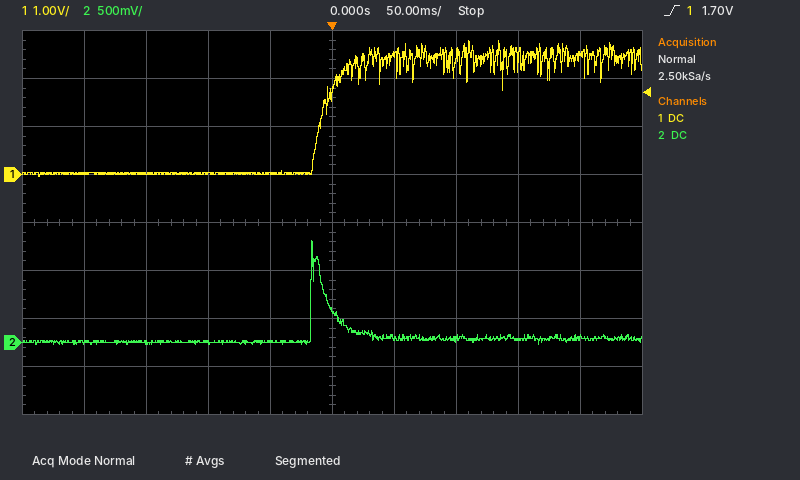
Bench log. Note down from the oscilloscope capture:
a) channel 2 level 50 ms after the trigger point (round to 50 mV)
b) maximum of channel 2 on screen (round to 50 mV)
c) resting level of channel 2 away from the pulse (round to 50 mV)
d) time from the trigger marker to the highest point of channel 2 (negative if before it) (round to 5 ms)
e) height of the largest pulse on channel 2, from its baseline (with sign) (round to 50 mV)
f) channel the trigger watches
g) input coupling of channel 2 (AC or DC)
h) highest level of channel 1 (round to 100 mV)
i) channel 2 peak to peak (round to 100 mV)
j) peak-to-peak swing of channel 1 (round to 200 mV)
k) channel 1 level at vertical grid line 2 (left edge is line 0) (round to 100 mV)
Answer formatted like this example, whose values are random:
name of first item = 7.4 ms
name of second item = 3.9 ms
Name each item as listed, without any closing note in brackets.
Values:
channel 2 level 50 ms after the trigger point = 50 mV
maximum of channel 2 on screen = 1.05 V
resting level of channel 2 away from the pulse = 0 mV
time from the trigger marker to the highest point of channel 2 (negative if before it) = -15 ms
height of the largest pulse on channel 2, from its baseline (with sign) = +1.05 V
channel the trigger watches = channel 1
input coupling of channel 2 = DC
highest level of channel 1 = 2.8 V
channel 2 peak to peak = 1.10 V
peak-to-peak swing of channel 1 = 2.8 V
channel 1 level at vertical grid line 2 (left edge is line 0) = 0.0 V
